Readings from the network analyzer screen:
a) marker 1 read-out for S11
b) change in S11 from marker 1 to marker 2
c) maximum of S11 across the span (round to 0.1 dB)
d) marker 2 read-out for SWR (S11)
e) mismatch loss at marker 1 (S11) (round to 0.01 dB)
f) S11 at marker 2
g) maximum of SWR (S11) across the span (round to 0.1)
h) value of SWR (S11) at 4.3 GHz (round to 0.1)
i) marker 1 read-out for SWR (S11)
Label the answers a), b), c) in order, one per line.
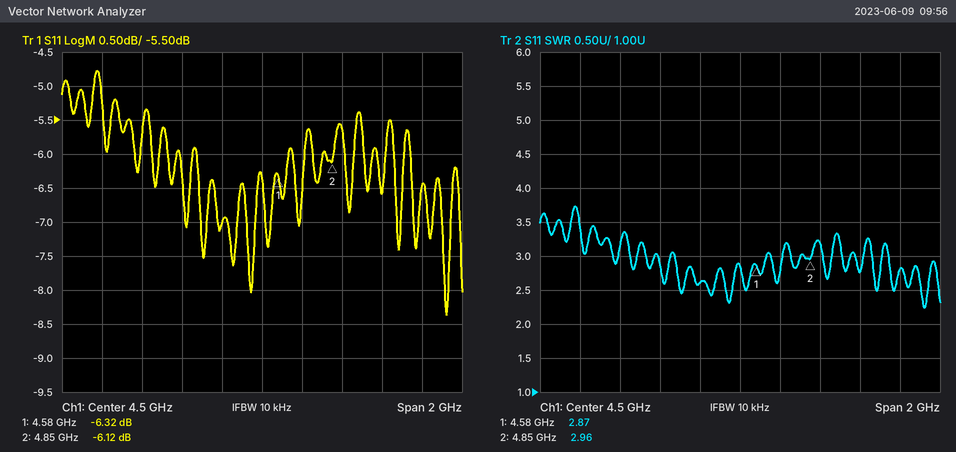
a) -6.32 dB
b) 0.20 dB
c) -4.8 dB
d) 2.96
e) 1.15 dB
f) -6.12 dB
g) 3.7
h) 2.6
i) 2.87
